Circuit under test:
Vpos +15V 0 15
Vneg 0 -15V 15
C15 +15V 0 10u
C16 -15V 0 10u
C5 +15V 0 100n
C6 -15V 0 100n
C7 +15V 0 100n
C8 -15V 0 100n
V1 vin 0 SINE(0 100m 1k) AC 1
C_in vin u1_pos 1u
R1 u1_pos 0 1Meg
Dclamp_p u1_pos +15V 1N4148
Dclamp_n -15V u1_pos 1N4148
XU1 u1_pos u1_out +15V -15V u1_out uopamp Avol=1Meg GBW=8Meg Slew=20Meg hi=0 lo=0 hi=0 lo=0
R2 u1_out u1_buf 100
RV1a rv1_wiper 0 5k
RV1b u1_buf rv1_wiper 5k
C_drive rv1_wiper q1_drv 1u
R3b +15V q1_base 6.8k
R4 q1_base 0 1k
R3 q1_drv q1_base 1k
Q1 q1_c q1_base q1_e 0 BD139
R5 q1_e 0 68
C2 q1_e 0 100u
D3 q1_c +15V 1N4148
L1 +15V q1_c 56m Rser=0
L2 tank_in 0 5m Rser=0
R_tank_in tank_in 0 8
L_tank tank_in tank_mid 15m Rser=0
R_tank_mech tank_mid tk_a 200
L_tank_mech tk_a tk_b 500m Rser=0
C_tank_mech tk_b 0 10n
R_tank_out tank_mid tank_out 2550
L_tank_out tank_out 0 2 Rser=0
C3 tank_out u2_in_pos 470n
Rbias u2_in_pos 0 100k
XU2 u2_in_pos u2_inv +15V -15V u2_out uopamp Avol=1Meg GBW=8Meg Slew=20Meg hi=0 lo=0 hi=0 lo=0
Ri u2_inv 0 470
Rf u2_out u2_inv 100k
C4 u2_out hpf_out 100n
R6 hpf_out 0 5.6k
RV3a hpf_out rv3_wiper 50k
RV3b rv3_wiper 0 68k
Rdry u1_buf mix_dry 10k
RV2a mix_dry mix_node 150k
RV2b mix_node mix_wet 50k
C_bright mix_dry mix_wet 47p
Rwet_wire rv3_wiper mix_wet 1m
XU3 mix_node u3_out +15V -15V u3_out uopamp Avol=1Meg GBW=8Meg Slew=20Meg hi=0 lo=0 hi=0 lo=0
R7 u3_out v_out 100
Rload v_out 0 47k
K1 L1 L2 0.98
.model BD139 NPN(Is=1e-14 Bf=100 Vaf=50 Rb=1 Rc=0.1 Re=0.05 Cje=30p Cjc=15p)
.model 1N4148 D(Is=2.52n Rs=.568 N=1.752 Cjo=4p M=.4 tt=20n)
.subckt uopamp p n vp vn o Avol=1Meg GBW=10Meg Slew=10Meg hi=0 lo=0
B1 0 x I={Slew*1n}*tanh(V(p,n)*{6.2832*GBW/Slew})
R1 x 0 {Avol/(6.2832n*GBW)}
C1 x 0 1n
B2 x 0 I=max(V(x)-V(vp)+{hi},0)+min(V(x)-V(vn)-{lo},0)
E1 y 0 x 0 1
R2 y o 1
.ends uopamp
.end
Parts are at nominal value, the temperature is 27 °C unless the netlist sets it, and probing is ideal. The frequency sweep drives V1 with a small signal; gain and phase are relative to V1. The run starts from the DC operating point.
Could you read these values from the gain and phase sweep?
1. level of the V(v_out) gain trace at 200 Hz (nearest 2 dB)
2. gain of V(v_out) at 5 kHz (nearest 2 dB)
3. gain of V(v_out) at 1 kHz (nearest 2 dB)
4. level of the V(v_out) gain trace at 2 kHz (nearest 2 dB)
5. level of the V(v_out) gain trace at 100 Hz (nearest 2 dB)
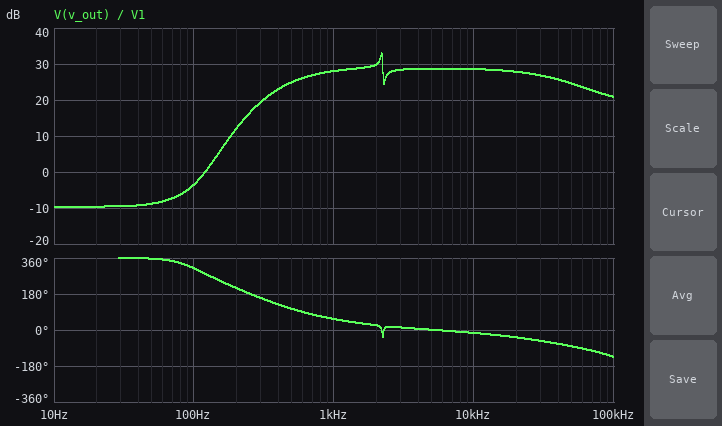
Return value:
12 dB
28 dB
28 dB
30 dB
-4 dB
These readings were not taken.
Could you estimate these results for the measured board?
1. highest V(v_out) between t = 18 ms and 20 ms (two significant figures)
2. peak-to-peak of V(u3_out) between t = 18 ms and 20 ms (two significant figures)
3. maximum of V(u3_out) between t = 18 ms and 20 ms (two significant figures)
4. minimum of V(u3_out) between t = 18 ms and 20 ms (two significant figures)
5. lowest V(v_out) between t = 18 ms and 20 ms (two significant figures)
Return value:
2.5 V
5.1 V
2.5 V
-2.5 V
-2.5 V
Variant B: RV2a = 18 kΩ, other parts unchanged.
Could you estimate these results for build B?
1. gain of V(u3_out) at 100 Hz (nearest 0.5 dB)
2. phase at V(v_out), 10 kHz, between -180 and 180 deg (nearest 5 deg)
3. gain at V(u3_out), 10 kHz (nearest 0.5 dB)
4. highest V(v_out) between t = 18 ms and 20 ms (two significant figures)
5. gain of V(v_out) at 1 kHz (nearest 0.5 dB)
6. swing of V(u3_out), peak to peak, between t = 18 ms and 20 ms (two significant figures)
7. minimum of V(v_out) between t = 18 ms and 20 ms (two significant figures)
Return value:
-2.0 dB
-10 deg
21.0 dB
1.0 V
20.5 dB
2.1 V
-1.0 V
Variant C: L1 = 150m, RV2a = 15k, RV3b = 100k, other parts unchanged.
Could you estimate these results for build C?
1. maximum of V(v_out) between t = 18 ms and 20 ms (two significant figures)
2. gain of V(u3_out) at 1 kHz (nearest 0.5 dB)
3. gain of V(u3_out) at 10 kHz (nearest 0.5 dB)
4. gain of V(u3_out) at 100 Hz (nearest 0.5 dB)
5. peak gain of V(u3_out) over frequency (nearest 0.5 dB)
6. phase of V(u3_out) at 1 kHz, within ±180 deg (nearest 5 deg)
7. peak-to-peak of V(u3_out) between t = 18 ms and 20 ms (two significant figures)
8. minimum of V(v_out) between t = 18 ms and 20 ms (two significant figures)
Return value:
1.7 V
24.5 dB
25.5 dB
-1.0 dB
30.0 dB
55 deg
3.4 V
-1.7 V
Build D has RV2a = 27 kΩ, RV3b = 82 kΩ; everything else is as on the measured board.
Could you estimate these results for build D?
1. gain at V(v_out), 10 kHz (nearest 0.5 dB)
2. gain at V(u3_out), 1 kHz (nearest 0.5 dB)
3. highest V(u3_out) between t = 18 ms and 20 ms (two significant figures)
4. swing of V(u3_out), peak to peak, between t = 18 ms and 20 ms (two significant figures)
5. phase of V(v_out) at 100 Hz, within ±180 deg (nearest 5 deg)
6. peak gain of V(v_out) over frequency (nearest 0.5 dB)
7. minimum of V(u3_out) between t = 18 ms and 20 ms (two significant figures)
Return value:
23.0 dB
22.5 dB
1.3 V
2.6 V
-20 deg
27.5 dB
-1.3 V
